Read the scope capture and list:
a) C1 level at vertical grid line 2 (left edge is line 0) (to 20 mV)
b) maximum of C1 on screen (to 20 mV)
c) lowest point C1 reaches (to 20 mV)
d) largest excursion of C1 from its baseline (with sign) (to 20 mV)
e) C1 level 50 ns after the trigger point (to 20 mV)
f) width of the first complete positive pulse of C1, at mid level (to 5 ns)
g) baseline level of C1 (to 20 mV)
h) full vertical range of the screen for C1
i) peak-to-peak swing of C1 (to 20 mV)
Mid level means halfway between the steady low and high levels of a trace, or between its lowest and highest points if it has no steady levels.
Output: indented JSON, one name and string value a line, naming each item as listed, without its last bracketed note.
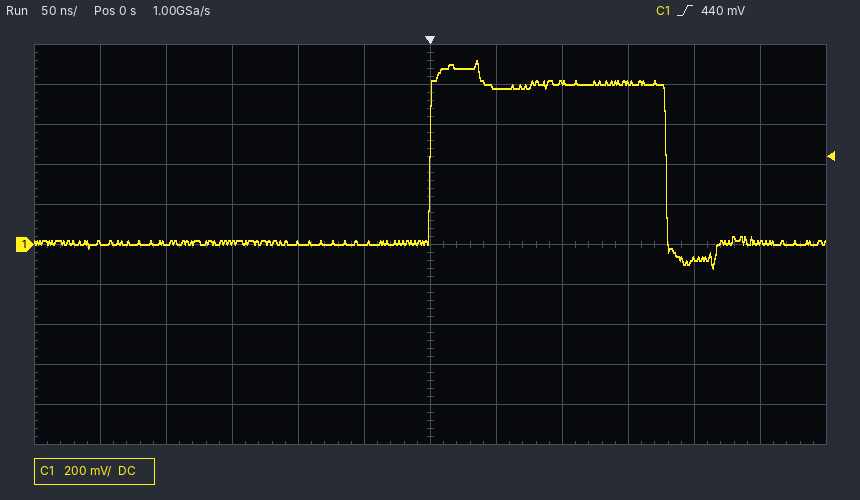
{
  "C1 level at vertical grid line 2 (left edge is line 0)": "0 mV",
  "maximum of C1 on screen": "920 mV",
  "lowest point C1 reaches": "-120 mV",
  "largest excursion of C1 from its baseline (with sign)": "+920 mV",
  "C1 level 50 ns after the trigger point": "780 mV",
  "width of the first complete positive pulse of C1, at mid level": "180 ns",
  "baseline level of C1": "0 mV",
  "full vertical range of the screen for C1": "2 V",
  "peak-to-peak swing of C1": "1.04 V"
}
